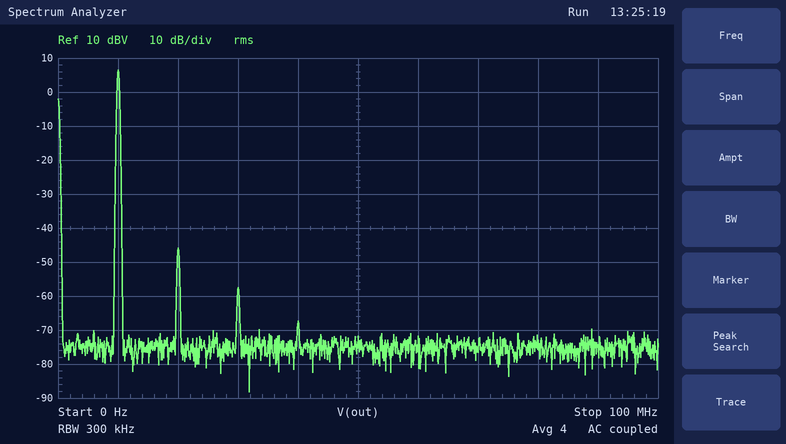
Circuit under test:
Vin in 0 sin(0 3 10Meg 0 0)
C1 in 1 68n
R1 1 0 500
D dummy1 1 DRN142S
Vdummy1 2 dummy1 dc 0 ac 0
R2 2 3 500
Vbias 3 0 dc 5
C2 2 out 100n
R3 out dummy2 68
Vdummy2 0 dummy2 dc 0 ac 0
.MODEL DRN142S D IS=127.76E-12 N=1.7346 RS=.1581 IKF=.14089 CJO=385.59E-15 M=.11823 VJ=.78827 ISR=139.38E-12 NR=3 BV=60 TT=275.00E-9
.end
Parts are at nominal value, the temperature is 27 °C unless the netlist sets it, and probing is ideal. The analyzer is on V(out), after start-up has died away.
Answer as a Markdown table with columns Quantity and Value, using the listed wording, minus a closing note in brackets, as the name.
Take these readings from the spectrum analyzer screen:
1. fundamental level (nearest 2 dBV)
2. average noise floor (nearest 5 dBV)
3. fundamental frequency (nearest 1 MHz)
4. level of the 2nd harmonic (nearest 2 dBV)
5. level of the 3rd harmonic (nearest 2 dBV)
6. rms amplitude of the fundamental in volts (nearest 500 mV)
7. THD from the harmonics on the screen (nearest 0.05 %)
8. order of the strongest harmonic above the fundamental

| Quantity | Value |
|---|---|
| fundamental level | 6 dBV |
| average noise floor | -75 dBV |
| fundamental frequency | 10 MHz |
| level of the 2nd harmonic | -46 dBV |
| level of the 3rd harmonic | -58 dBV |
| rms amplitude of the fundamental in volts | 2.0 V |
| THD from the harmonics on the screen | 0.25 % |
| order of the strongest harmonic above the fundamental | 2 |
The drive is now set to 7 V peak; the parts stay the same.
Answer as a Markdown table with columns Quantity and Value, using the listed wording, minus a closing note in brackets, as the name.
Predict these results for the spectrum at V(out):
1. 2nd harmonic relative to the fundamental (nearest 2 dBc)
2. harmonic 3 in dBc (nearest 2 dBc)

| Quantity | Value |
|---|---|
| 2nd harmonic relative to the fundamental | -16 dBc |
| harmonic 3 in dBc | -18 dBc |
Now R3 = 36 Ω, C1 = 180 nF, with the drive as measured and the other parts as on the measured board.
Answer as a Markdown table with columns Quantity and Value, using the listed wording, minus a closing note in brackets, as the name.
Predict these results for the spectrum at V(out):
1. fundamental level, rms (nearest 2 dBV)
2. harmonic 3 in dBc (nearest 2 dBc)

| Quantity | Value |
|---|---|
| fundamental level, rms | 6 dBV |
| harmonic 3 in dBc | -22 dBc |
